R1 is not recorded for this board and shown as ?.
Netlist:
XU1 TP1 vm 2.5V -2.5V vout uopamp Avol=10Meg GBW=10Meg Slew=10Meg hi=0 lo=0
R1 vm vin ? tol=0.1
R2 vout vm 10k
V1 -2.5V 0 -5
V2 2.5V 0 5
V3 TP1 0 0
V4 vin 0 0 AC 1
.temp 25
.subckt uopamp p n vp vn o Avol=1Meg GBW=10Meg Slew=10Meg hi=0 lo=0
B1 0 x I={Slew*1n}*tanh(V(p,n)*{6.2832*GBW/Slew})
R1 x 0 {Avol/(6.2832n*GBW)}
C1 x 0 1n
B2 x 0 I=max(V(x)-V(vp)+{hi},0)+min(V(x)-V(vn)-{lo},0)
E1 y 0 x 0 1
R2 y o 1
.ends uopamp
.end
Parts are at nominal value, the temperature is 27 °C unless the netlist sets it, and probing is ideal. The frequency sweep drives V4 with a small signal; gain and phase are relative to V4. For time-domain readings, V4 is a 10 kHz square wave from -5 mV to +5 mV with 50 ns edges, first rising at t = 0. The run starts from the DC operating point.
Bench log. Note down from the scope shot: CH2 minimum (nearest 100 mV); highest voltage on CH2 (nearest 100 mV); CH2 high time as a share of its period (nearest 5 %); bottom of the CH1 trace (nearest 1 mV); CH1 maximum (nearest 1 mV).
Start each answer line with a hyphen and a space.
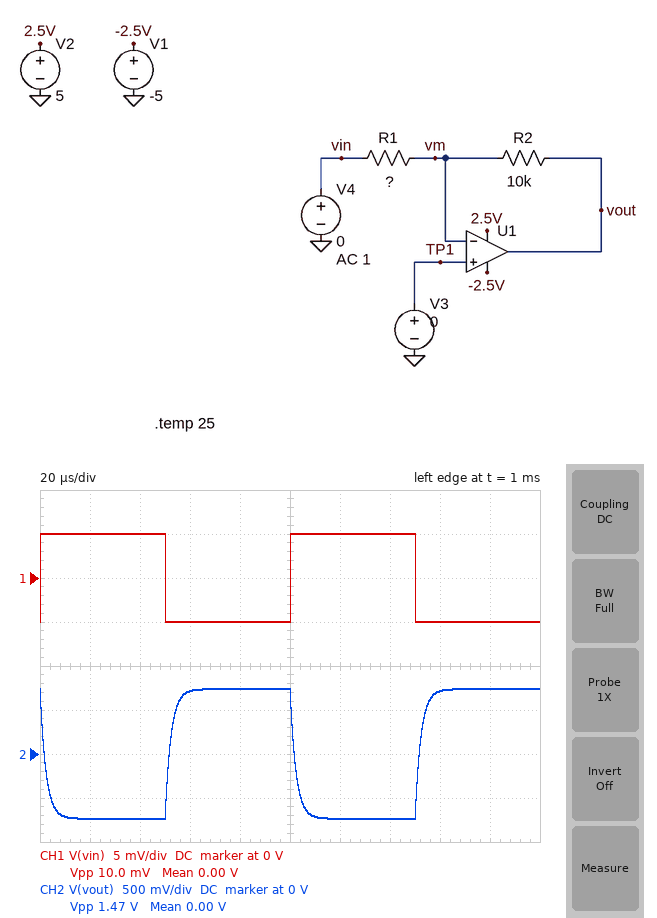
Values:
- -700 mV
- 700 mV
- 50 %
- -5 mV
- 5 mV
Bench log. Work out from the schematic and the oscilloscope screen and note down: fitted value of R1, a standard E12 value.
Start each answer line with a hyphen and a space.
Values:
- 68 Ω
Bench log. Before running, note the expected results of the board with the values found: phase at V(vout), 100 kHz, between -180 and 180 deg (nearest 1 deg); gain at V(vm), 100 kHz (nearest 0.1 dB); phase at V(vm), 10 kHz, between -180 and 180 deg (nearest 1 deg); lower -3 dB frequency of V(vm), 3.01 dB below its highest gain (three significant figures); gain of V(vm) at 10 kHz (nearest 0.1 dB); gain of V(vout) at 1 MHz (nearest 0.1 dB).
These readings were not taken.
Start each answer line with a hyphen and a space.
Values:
- 124 deg
- -1.7 dB
- 82 deg
- 67.5 kHz
- -16.7 dB
- 19.9 dB
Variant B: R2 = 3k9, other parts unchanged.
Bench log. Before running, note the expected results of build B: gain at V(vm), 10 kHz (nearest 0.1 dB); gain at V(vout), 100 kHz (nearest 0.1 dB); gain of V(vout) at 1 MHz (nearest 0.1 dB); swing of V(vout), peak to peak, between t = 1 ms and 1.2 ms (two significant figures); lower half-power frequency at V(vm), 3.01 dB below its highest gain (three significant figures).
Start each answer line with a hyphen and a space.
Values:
- -24.8 dB
- 33.9 dB
- 19.7 dB
- 570 mV
- 171 kHz
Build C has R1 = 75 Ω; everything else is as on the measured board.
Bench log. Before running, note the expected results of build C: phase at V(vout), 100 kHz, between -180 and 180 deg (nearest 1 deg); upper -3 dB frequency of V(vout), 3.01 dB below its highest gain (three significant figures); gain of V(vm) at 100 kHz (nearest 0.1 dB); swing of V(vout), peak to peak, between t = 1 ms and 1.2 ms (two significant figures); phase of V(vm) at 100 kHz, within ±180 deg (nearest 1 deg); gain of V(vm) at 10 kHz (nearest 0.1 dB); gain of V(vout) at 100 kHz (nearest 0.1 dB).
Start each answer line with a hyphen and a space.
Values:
- 127 deg
- 74.4 kHz
- -2.0 dB
- 1.3 V
- 37 deg
- -17.6 dB
- 38.0 dB
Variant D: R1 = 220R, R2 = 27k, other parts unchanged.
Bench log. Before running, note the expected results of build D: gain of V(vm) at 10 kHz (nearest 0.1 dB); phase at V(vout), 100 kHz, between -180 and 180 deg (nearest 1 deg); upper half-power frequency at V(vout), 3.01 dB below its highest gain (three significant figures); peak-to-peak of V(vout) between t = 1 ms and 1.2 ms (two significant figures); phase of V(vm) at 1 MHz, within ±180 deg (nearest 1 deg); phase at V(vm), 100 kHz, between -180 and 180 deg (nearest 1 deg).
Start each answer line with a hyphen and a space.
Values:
- -18.3 dB
- 129 deg
- 80.8 kHz
- 1.2 V
- 5 deg
- 39 deg
